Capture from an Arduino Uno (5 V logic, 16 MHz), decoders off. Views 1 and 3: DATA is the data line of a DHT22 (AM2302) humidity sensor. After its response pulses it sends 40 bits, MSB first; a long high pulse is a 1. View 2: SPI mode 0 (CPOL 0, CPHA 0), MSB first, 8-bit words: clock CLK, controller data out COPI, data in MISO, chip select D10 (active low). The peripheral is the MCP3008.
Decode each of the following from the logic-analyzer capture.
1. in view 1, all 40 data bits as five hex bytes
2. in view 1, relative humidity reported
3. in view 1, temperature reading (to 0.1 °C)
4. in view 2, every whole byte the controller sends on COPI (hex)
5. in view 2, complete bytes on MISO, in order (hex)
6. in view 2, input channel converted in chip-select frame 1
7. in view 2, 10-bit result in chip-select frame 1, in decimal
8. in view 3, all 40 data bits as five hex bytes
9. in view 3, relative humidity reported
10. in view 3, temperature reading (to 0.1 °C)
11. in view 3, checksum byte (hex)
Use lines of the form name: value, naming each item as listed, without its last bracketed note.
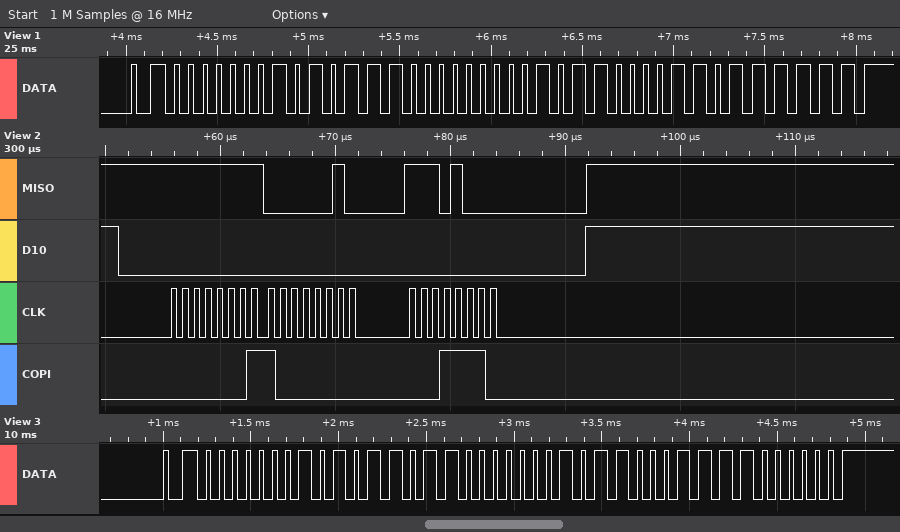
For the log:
in view 1, all 40 data bits as five hex bytes: 01 5C 01 61 BF
in view 1, relative humidity reported: 34.8 %
in view 1, temperature reading: 35.3 °C
in view 2, every whole byte the controller sends on COPI: 01 80 1E
in view 2, complete bytes on MISO, in order: FF 02 E8
in view 2, input channel converted in chip-select frame 1: 0
in view 2, 10-bit result in chip-select frame 1, in decimal: 744
in view 3, all 40 data bits as five hex bytes: 01 5B 01 63 C0
in view 3, relative humidity reported: 34.7 %
in view 3, temperature reading: 35.5 °C
in view 3, checksum byte: 0xC0
